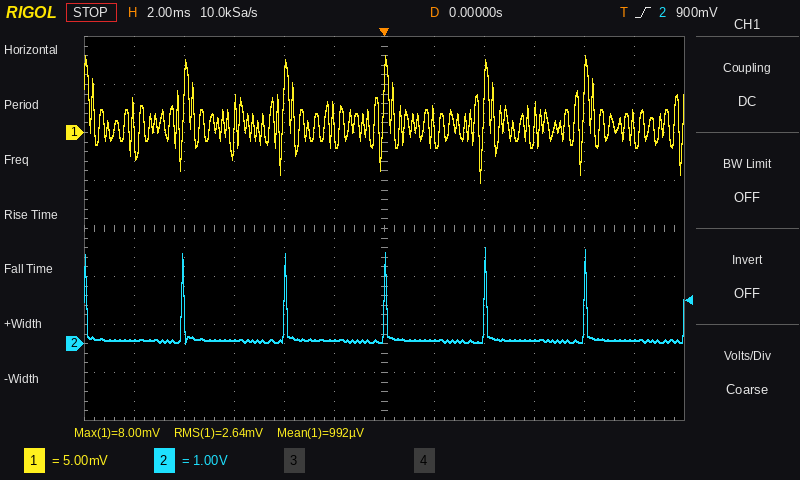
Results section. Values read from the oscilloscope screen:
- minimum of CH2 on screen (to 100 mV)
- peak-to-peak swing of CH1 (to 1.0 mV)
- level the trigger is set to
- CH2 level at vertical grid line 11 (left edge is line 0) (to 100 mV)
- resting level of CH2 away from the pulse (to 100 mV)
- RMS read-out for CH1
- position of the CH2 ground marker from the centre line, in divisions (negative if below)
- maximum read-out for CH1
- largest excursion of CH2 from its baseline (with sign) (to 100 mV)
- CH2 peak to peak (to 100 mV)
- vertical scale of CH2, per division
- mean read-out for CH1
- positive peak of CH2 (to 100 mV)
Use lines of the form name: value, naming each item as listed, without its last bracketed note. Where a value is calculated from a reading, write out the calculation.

minimum of CH2 on screen: 0.0 V
peak-to-peak swing of CH1: 13.0 mV
level the trigger is set to: 900 mV
CH2 level at vertical grid line 11 (left edge is line 0): 100 mV
resting level of CH2 away from the pulse: 100 mV
RMS read-out for CH1: 2.64 mV
position of the CH2 ground marker from the centre line, in divisions: -2.4 div
maximum read-out for CH1: 8.00 mV
largest excursion of CH2 from its baseline (with sign): 2.0 V − (100 mV) = +1.9 V
CH2 peak to peak: 2.0 V − (0.0 V) = 2.0 V
vertical scale of CH2, per division: 1 V
mean read-out for CH1: 992 µV
positive peak of CH2: 2.0 V
